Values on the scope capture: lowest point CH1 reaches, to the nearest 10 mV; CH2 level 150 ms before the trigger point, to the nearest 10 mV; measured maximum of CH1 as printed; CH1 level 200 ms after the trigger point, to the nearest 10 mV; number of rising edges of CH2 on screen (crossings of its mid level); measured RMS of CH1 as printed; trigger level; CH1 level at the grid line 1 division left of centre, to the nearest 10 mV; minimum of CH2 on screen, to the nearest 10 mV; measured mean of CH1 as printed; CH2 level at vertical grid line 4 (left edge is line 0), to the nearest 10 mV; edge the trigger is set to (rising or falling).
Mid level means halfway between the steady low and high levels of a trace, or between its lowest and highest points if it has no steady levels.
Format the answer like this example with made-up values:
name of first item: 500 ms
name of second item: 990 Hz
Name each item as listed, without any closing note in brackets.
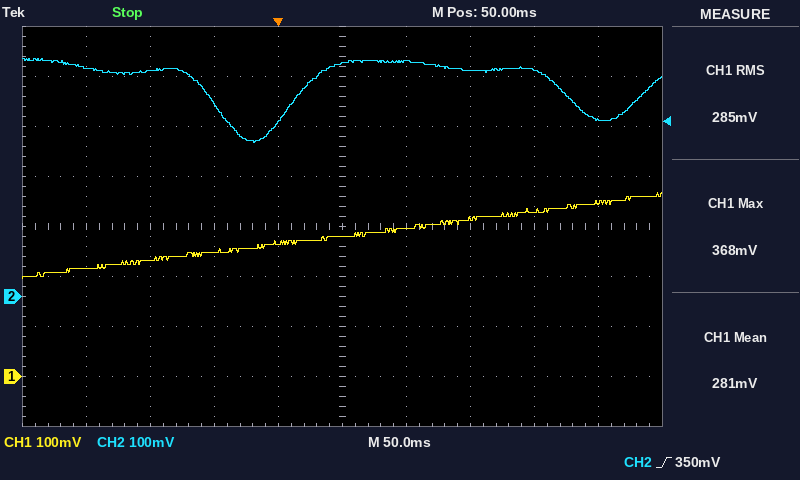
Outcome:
lowest point CH1 reaches, to the nearest 10 mV: 200 mV
CH2 level 150 ms before the trigger point, to the nearest 10 mV: 460 mV
measured maximum of CH1 as printed: 368 mV
CH1 level 200 ms after the trigger point, to the nearest 10 mV: 330 mV
number of rising edges of CH2 on screen: 2
measured RMS of CH1 as printed: 285 mV
trigger level: 350 mV
CH1 level at the grid line 1 division left of centre, to the nearest 10 mV: 270 mV
minimum of CH2 on screen, to the nearest 10 mV: 310 mV
measured mean of CH1 as printed: 281 mV
CH2 level at vertical grid line 4 (left edge is line 0), to the nearest 10 mV: 350 mV
edge the trigger is set to: rising
